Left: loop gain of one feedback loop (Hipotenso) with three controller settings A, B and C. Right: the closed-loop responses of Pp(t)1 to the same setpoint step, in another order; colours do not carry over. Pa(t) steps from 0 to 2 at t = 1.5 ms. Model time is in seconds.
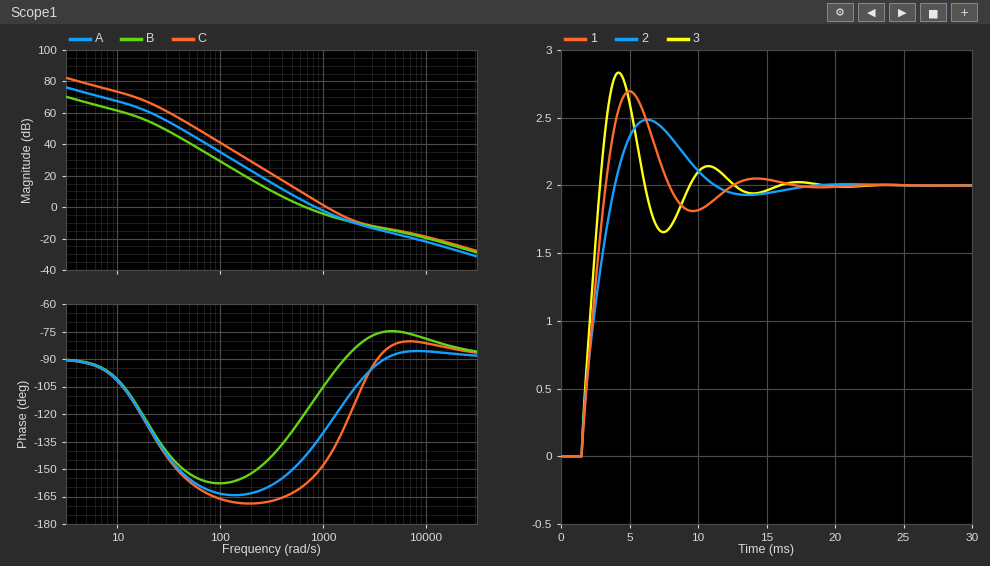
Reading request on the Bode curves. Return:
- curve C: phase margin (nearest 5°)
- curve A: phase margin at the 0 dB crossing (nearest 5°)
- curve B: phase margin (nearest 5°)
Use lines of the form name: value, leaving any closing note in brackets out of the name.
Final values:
curve C: phase margin: 35°
curve A: phase margin at the 0 dB crossing: 45°
curve B: phase margin: 60°
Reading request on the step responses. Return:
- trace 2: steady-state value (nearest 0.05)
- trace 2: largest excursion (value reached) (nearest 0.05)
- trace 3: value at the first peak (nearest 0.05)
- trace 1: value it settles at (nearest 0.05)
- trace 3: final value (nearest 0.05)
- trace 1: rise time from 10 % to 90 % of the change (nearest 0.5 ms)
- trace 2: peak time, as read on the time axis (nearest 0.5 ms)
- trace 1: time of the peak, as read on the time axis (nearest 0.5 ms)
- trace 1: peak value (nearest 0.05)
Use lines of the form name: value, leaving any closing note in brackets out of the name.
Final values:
trace 2: steady-state value: 2.00
trace 2: largest excursion (value reached): 2.50
trace 3: value at the first peak: 2.85
trace 1: value it settles at: 2.00
trace 3: final value: 2.00
trace 1: rise time from 10 % to 90 % of the change: 1.5 ms
trace 2: peak time, as read on the time axis: 6.5 ms
trace 1: time of the peak, as read on the time axis: 5.0 ms
trace 1: peak value: 2.70
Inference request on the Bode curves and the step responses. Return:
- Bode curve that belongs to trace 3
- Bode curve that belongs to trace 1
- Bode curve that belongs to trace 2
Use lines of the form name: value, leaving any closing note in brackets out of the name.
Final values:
Bode curve that belongs to trace 3: C
Bode curve that belongs to trace 1: A
Bode curve that belongs to trace 2: B
